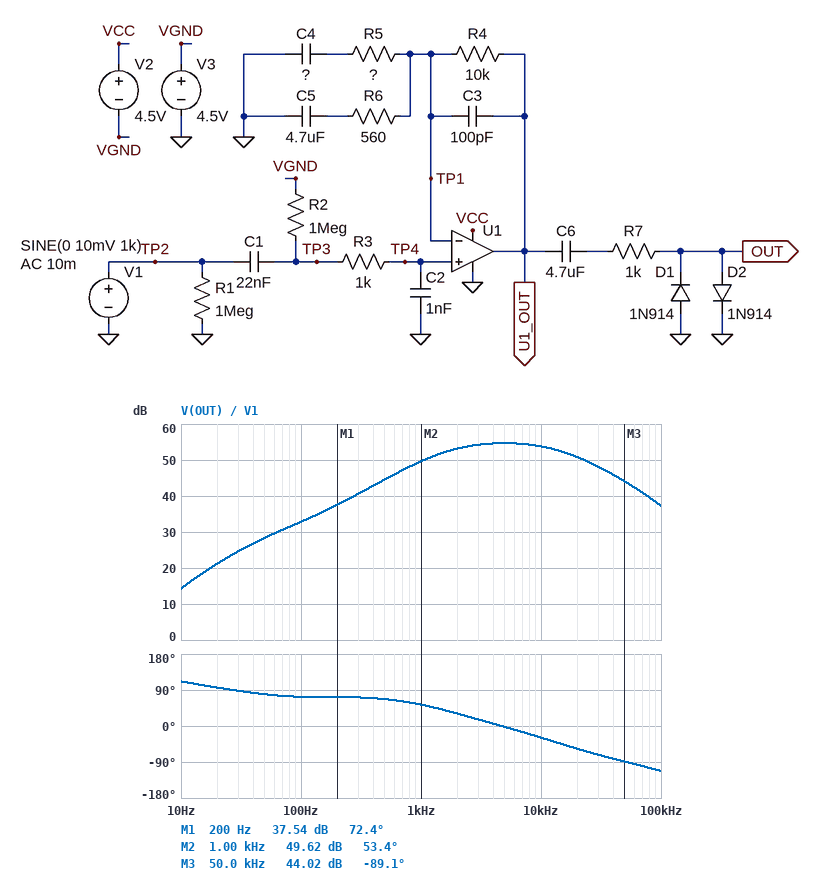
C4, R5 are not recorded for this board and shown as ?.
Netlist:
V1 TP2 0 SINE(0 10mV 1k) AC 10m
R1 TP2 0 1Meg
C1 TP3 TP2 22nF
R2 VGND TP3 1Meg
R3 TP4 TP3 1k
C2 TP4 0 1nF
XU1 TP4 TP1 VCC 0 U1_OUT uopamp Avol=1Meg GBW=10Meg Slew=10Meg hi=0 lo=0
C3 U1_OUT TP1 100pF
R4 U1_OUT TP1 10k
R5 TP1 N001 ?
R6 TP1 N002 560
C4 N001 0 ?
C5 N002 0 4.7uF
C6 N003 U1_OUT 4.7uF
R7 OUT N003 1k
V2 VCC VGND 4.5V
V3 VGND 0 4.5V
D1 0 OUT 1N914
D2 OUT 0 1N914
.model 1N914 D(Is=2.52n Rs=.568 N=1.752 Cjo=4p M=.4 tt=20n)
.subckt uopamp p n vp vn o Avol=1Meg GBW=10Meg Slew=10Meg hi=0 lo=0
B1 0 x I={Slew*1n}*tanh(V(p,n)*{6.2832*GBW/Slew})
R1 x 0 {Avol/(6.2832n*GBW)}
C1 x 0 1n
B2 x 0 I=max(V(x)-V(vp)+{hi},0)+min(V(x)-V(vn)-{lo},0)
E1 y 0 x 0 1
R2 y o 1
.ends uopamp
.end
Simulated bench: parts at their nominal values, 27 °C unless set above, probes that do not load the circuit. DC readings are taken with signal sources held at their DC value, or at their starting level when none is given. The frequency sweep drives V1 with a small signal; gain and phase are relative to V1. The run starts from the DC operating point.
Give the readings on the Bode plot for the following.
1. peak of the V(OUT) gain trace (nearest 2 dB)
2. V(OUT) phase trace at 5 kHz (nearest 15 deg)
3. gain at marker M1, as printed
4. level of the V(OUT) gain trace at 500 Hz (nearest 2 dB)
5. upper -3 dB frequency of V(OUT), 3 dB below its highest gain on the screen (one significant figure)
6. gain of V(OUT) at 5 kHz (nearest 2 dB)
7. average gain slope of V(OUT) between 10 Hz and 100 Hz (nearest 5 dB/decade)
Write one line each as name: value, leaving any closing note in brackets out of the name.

peak of the V(OUT) gain trace: 54 dB
V(OUT) phase trace at 5 kHz: 0 deg
gain at marker M1, as printed: 37.54 dB
level of the V(OUT) gain trace at 500 Hz: 44 dB
upper -3 dB frequency of V(OUT), 3 dB below its highest gain on the screen: 20 kHz
gain of V(OUT) at 5 kHz: 54 dB
average gain slope of V(OUT) between 10 Hz and 100 Hz: 20 dB/decade
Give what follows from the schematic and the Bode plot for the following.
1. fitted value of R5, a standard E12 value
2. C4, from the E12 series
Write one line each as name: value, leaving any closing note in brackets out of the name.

fitted value of R5, a standard E12 value: 18 Ω
C4, from the E12 series: 5.6 µF
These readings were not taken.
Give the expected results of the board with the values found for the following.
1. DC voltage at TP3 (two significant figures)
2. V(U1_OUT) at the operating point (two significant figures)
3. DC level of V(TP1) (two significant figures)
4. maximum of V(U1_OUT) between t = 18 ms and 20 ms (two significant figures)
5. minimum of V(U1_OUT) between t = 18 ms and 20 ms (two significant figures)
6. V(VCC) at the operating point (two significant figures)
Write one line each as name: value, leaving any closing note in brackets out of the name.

DC voltage at TP3: 4.5 V
V(U1_OUT) at the operating point: 4.5 V
DC level of V(TP1): 4.5 V
maximum of V(U1_OUT) between t = 18 ms and 20 ms: 7.5 V
minimum of V(U1_OUT) between t = 18 ms and 20 ms: 1.5 V
V(VCC) at the operating point: 9.0 V
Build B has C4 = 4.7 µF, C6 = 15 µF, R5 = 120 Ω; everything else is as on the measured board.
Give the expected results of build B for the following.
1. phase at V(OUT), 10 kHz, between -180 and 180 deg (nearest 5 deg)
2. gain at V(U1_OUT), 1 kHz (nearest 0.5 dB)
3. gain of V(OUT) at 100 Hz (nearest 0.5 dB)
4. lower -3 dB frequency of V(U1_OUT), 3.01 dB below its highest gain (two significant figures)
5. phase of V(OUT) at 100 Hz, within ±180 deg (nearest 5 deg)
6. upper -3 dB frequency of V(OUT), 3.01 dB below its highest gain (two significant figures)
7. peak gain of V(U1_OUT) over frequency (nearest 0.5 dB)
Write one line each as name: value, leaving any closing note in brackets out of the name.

phase at V(OUT), 10 kHz, between -180 and 180 deg: -10 deg
gain at V(U1_OUT), 1 kHz: 39.5 dB
gain of V(OUT) at 100 Hz: 32.0 dB
lower -3 dB frequency of V(U1_OUT), 3.01 dB below its highest gain: 260 Hz
phase of V(OUT) at 100 Hz, within ±180 deg: 60 deg
upper -3 dB frequency of V(OUT), 3.01 dB below its highest gain: 55 kHz
peak gain of V(U1_OUT) over frequency: 40.0 dB
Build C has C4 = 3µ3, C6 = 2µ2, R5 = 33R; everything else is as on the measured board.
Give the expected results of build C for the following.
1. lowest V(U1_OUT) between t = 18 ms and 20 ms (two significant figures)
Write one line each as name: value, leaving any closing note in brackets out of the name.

lowest V(U1_OUT) between t = 18 ms and 20 ms: 2.7 V
